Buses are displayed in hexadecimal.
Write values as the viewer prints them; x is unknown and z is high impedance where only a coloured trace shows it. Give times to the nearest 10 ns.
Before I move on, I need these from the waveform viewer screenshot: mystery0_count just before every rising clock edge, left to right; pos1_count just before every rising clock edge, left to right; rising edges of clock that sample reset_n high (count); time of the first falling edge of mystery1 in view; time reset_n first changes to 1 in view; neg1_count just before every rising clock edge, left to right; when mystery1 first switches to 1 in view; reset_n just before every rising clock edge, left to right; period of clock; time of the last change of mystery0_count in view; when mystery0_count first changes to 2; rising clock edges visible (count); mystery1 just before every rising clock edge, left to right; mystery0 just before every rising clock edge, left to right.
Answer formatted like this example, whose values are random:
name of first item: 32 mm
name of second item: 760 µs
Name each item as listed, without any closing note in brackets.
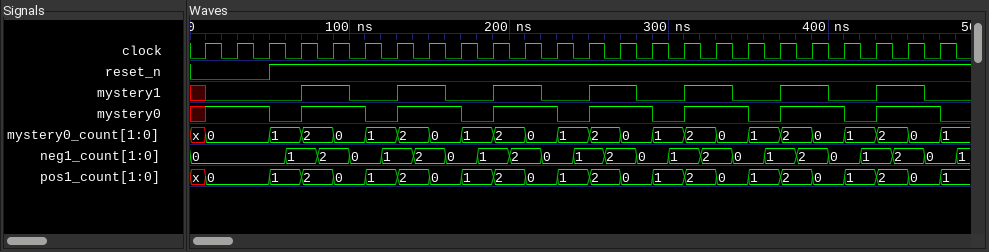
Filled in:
mystery0_count just before every rising clock edge, left to right: x, 0, 0, 1, 2, 0, 1, 2, 0, 1, 2, 0, 1, 2, 0, 1, 2, 0, 1, 2, 0, 1, 2, 0
pos1_count just before every rising clock edge, left to right: x, 0, 0, 1, 2, 0, 1, 2, 0, 1, 2, 0, 1, 2, 0, 1, 2, 0, 1, 2, 0, 1, 2, 0
rising edges of clock that sample reset_n high: 21
time of the first falling edge of mystery1 in view: 100 ns
time reset_n first changes to 1 in view: 50 ns
neg1_count just before every rising clock edge, left to right: 0, 0, 0, 1, 2, 0, 1, 2, 0, 1, 2, 0, 1, 2, 0, 1, 2, 0, 1, 2, 0, 1, 2, 0
when mystery1 first switches to 1 in view: 70 ns
reset_n just before every rising clock edge, left to right: 0 0 0 1 1 1 1 1 1 1 1 1 1 1 1 1 1 1 1 1 1 1 1 1
period of clock: 20 ns
time of the last change of mystery0_count in view: 470 ns
when mystery0_count first changes to 2: 70 ns
rising clock edges visible: 24
mystery1 just before every rising clock edge, left to right: x 0 0 0 1 0 0 1 0 0 1 0 0 1 0 0 1 0 0 1 0 0 1 0
mystery0 just before every rising clock edge, left to right: x 1 1 0 1 1 0 1 1 0 1 1 0 1 1 0 1 1 0 1 1 0 1 1
